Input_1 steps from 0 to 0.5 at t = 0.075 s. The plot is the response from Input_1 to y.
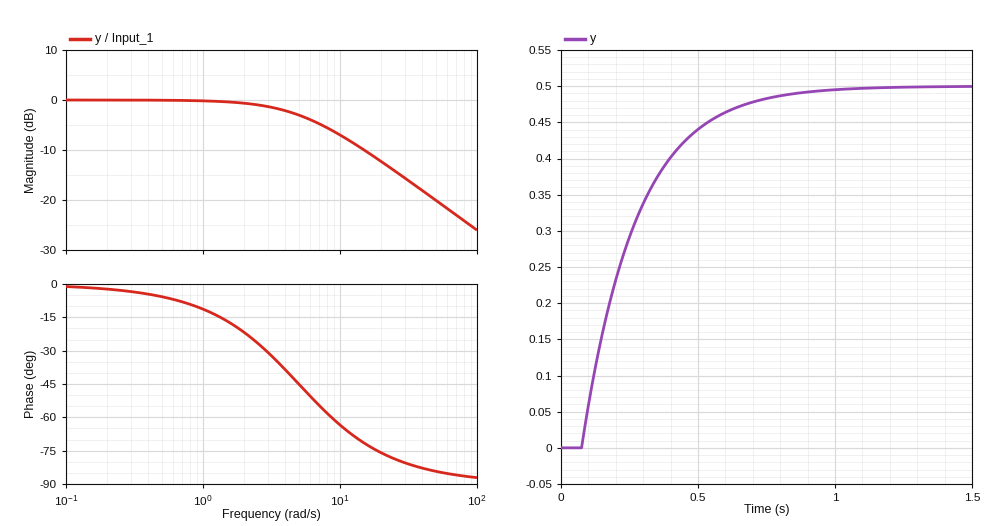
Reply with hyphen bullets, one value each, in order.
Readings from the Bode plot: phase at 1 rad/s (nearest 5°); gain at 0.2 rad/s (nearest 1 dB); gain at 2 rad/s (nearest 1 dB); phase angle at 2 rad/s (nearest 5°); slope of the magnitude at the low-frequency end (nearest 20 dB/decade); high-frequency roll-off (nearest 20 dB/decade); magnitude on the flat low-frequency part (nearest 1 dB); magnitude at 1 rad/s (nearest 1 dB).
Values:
- -10°
- 0 dB
- -1 dB
- -20°
- 0 dB/decade
- -20 dB/decade
- 0 dB
- 0 dB
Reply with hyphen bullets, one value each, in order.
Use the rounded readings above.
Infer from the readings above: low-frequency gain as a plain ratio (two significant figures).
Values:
- 1.0
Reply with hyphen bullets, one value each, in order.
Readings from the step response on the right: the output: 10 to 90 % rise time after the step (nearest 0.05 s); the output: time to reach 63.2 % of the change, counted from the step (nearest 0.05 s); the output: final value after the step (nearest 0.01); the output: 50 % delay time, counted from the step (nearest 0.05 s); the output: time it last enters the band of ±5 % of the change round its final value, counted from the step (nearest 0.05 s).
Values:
- 0.45 s
- 0.20 s
- 0.50
- 0.15 s
- 0.60 s
